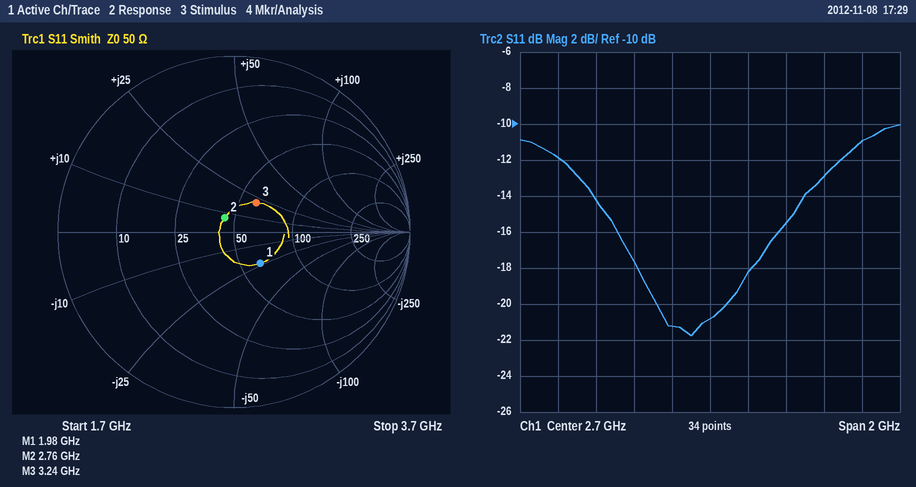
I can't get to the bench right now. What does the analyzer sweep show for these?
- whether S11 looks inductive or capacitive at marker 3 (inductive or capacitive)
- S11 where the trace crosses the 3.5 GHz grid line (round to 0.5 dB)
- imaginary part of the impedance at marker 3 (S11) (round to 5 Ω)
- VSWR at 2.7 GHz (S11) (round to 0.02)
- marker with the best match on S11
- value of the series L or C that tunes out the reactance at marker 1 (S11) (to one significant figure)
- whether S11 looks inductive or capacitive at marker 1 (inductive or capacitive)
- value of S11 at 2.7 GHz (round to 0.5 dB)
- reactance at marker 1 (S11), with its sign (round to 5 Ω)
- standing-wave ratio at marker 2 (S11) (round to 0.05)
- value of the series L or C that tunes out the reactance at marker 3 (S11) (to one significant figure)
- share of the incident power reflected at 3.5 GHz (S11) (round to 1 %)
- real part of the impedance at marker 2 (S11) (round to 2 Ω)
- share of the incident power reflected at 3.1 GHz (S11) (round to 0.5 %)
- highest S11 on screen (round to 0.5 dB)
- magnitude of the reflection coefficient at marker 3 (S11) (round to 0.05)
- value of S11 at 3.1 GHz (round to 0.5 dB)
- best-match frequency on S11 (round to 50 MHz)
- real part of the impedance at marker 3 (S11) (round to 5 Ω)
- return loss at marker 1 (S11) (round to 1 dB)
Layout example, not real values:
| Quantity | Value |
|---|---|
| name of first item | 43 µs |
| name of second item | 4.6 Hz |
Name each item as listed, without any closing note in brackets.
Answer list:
| Quantity | Value |
|---|---|
| whether S11 looks inductive or capacitive at marker 3 | inductive |
| S11 where the trace crosses the 3.5 GHz grid line | -11.0 dB |
| imaginary part of the impedance at marker 3 (S11) | +20 Ω |
| VSWR at 2.7 GHz (S11) | 1.20 |
| marker with the best match on S11 | marker 2 |
| value of the series L or C that tunes out the reactance at marker 1 (S11) | 2 nH |
| whether S11 looks inductive or capacitive at marker 1 | capacitive |
| value of S11 at 2.7 GHz | -21.0 dB |
| reactance at marker 1 (S11), with its sign | -25 Ω |
| standing-wave ratio at marker 2 (S11) | 1.20 |
| value of the series L or C that tunes out the reactance at marker 3 (S11) | 2 pF |
| share of the incident power reflected at 3.5 GHz (S11) | 8 % |
| real part of the impedance at marker 2 (S11) | 44 Ω |
| share of the incident power reflected at 3.1 GHz (S11) | 3.0 % |
| highest S11 on screen | -10.0 dB |
| magnitude of the reflection coefficient at marker 3 (S11) | 0.20 |
| value of S11 at 3.1 GHz | -15.5 dB |
| best-match frequency on S11 | 2.60 GHz |
| real part of the impedance at marker 3 (S11) | 60 Ω |
| return loss at marker 1 (S11) | 13 dB |
